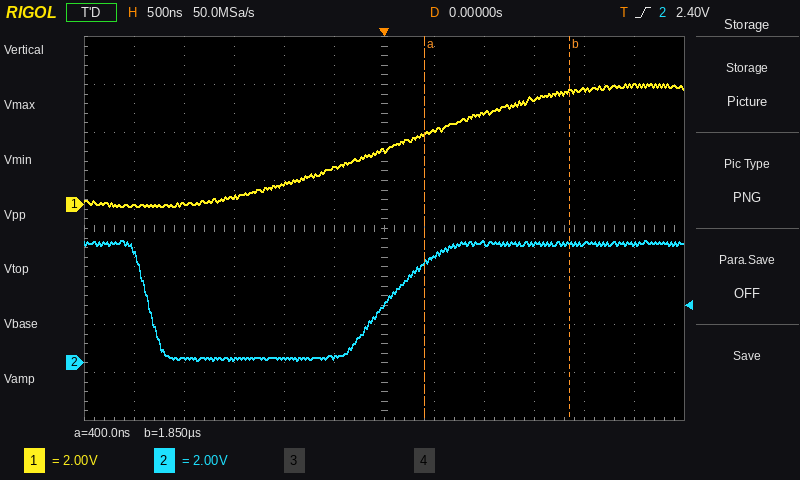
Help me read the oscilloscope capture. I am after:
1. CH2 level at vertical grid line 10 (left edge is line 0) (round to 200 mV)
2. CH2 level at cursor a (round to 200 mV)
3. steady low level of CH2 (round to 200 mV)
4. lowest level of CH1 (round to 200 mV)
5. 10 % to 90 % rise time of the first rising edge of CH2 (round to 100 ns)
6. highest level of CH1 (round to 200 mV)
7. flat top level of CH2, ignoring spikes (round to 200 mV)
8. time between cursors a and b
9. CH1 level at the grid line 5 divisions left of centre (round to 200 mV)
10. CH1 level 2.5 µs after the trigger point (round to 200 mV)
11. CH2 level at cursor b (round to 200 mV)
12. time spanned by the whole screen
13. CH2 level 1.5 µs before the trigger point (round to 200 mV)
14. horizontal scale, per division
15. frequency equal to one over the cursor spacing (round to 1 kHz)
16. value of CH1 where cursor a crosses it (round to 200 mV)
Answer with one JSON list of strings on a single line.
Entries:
["5.0 V", "4.2 V", "200 mV", "0.0 V", "800 ns", "5.0 V", "5.0 V", "1.45 µs", "0.0 V", "5.0 V", "5.0 V", "6 µs", "200 mV", "500 ns", "690 kHz", "3.0 V"]
